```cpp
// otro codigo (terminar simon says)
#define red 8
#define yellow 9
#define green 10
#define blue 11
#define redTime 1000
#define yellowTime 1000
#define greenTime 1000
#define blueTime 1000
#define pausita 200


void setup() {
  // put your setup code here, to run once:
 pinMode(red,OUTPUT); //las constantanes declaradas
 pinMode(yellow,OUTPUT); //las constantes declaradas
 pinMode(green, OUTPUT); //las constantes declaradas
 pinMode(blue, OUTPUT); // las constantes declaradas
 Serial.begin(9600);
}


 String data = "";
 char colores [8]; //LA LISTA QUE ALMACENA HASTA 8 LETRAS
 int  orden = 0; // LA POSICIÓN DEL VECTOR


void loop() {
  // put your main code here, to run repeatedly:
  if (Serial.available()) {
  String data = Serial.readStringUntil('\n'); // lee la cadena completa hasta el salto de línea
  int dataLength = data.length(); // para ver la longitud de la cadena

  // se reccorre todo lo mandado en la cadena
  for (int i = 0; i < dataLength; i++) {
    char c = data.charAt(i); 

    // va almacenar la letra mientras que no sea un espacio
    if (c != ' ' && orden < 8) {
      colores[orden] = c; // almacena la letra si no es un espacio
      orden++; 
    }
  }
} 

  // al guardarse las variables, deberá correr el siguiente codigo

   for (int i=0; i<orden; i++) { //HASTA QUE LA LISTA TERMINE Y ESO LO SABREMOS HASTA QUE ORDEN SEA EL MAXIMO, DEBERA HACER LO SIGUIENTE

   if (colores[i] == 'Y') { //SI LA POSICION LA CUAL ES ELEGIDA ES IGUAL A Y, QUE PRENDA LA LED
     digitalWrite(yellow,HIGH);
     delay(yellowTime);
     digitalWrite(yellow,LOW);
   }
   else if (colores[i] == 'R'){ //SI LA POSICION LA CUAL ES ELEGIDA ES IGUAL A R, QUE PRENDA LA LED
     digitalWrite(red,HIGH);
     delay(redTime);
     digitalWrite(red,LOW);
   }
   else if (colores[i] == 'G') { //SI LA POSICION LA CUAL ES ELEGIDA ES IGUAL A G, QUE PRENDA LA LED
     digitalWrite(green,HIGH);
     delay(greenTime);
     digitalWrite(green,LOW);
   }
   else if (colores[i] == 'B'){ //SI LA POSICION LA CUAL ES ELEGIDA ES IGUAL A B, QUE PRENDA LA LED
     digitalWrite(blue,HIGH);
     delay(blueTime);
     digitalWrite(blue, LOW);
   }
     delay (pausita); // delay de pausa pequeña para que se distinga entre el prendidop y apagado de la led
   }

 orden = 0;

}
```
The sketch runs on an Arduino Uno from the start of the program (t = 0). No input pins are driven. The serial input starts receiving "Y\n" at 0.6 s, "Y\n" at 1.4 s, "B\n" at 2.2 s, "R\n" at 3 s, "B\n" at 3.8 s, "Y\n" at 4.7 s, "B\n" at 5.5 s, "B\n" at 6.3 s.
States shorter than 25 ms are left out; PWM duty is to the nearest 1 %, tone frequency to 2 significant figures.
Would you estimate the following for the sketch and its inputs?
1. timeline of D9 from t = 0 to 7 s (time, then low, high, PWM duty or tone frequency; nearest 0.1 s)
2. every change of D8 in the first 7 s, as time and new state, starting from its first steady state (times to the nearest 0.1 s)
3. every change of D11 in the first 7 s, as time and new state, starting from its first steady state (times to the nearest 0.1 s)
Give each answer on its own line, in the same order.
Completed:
0 s low; 0.6 s high; 1.6 s low; 1.8 s high; 2.8 s low; 6.6 s high
0 s low; 4.2 s high; 5.2 s low
0 s low; 3 s high; 4 s low; 5.4 s high; 6.4 s low
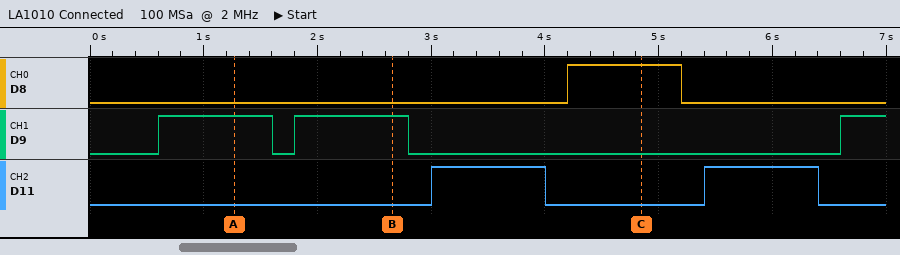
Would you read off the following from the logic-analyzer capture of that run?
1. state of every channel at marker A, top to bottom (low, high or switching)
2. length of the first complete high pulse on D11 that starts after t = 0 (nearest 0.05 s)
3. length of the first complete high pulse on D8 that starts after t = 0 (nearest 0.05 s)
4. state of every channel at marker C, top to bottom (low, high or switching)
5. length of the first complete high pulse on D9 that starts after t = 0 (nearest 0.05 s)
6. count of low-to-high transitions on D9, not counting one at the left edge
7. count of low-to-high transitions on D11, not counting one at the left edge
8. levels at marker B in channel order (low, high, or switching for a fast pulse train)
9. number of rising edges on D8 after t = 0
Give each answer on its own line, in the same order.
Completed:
D8 low, D9 high, D11 low
1.00 s
1.00 s
D8 high, D9 low, D11 low
1.00 s
3
2
D8 low, D9 high, D11 low
1
